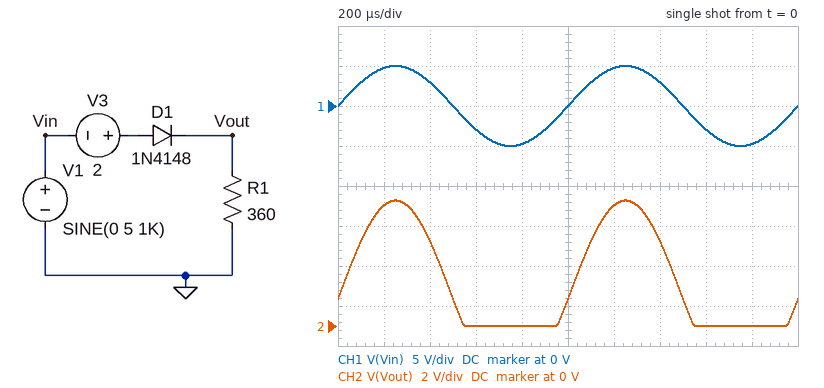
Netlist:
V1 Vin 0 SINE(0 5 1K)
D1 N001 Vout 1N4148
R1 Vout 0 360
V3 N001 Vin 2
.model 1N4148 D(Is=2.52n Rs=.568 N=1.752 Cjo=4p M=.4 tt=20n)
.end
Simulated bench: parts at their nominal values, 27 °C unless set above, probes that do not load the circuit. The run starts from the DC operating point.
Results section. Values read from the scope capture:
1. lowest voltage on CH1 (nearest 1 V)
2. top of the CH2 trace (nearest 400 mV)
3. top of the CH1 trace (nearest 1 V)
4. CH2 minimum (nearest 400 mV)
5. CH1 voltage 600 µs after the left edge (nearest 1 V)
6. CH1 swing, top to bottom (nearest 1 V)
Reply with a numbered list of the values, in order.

1. -5 V
2. 6.4 V
3. 5 V
4. 0 V
5. -3 V
6. 10 V
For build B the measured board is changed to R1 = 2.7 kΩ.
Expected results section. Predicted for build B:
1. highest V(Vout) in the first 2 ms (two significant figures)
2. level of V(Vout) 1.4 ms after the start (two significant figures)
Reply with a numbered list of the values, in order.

1. 6.4 V
2. 4.3 V
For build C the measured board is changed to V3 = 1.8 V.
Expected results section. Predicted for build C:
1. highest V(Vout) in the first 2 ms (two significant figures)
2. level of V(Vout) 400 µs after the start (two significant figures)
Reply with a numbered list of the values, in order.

1. 6.1 V
2. 4.0 V
